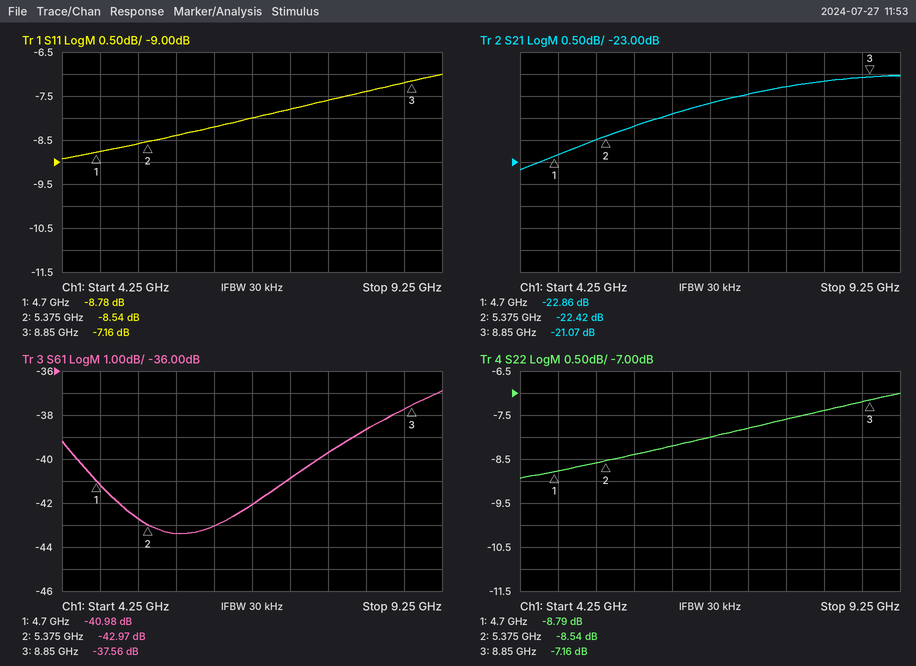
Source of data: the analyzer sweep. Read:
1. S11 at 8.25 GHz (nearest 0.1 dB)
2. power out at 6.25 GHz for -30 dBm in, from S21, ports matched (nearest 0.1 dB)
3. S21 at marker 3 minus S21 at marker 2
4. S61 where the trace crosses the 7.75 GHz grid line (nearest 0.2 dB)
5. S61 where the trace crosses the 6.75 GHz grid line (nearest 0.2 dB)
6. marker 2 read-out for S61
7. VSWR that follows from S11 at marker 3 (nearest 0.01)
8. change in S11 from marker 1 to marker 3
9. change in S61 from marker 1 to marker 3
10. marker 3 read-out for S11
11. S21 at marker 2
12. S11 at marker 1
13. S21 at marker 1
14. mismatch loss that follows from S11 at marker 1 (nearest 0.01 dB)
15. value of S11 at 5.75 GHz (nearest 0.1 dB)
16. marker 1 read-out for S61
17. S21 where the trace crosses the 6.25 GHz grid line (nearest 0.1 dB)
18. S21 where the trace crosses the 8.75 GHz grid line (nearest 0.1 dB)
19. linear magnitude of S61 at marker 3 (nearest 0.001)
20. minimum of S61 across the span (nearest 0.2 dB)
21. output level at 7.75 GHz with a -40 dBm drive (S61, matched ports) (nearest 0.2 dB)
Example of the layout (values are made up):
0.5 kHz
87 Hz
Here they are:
-7.4 dB
-51.9 dBm
1.35 dB
-39.8 dB
-42.0 dB
-42.97 dB
2.56
1.62 dB
3.42 dB
-7.16 dB
-22.42 dB
-8.78 dB
-22.86 dB
0.62 dB
-8.4 dB
-40.98 dB
-21.9 dB
-21.1 dB
0.013
-43.4 dB
-79.8 dBm
